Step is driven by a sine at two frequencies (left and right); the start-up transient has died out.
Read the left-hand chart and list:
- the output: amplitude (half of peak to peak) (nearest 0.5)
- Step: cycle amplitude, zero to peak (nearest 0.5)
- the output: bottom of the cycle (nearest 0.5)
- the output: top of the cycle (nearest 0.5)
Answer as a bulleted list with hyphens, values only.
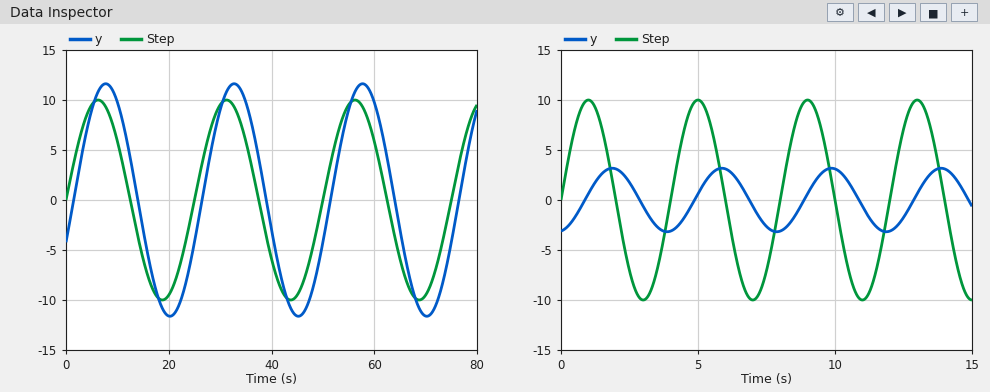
- 11.5
- 10.0
- -11.5
- 11.5
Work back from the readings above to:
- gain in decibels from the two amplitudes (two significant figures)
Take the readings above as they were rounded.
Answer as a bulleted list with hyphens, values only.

- 1.2 dB
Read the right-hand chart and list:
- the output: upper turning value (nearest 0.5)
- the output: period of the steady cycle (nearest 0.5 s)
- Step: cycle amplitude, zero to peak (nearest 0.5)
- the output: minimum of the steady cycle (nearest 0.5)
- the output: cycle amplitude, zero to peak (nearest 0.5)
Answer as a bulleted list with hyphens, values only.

- 3.0
- 4.0 s
- 10.0
- -3.0
- 3.0
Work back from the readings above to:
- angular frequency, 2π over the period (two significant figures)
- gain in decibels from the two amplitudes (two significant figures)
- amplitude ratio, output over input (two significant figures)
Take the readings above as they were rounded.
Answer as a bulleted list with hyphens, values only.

- 1.6 rad/s
- -10 dB
- 0.30
